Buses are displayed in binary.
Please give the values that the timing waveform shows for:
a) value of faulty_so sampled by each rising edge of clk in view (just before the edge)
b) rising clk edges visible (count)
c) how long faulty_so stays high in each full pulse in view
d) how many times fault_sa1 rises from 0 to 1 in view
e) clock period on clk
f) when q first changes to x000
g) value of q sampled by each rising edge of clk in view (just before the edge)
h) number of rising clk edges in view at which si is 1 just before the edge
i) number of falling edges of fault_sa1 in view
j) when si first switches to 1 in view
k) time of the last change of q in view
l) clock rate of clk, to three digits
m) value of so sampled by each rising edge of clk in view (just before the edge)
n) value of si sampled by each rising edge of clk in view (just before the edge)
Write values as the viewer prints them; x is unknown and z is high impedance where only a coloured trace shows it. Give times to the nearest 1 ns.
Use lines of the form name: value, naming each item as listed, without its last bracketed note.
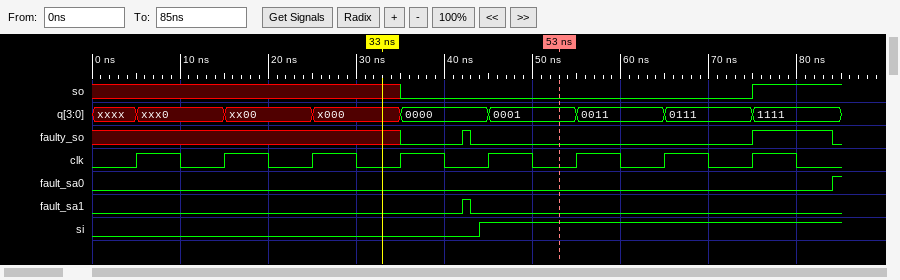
value of faulty_so sampled by each rising edge of clk in view: x x x x 0 0 0 0
rising clk edges visible: 8
how long faulty_so stays high in each full pulse in view: 1 ns, 9 ns
how many times fault_sa1 rises from 0 to 1 in view: 1
clock period on clk: 10 ns
when q first changes to x000: 25 ns
value of q sampled by each rising edge of clk in view: xxxx, xxx0, xx00, x000, 0000, 0001, 0011, 0111
number of rising clk edges in view at which si is 1 just before the edge: 4
number of falling edges of fault_sa1 in view: 1
when si first switches to 1 in view: 44 ns
time of the last change of q in view: 75 ns
clock rate of clk, to three digits: 100 MHz
value of so sampled by each rising edge of clk in view: x x x x 0 0 0 0
value of si sampled by each rising edge of clk in view: 0 0 0 0 1 1 1 1
